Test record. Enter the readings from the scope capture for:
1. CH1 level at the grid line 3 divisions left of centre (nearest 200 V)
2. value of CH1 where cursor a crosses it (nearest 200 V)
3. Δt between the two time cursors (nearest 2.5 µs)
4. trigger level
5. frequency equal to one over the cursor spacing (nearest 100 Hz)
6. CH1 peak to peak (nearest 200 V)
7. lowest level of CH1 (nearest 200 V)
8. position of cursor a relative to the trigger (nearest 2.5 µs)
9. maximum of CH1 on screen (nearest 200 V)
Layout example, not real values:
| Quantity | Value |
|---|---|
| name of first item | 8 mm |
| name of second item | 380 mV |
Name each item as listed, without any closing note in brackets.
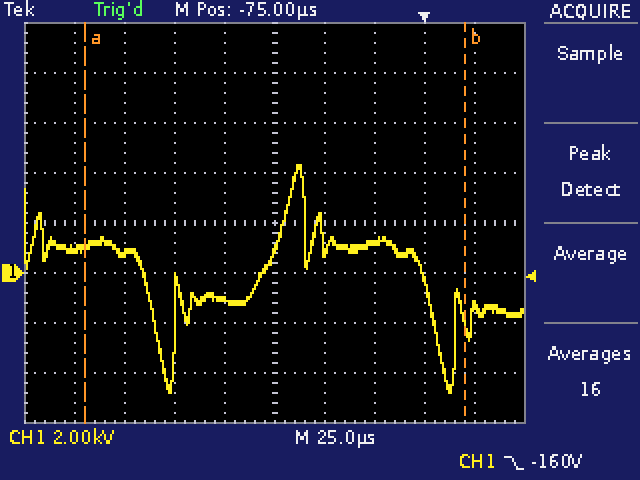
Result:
| Quantity | Value |
|---|---|
| CH1 level at the grid line 3 divisions left of centre | 800 V |
| value of CH1 where cursor a crosses it | 1.0 kV |
| Δt between the two time cursors | 190.0 µs |
| trigger level | -160 V |
| frequency equal to one over the cursor spacing | 5.3 kHz |
| CH1 peak to peak | 9.2 kV |
| lowest level of CH1 | -4.8 kV |
| position of cursor a relative to the trigger | -170.0 µs |
| maximum of CH1 on screen | 4.4 kV |
